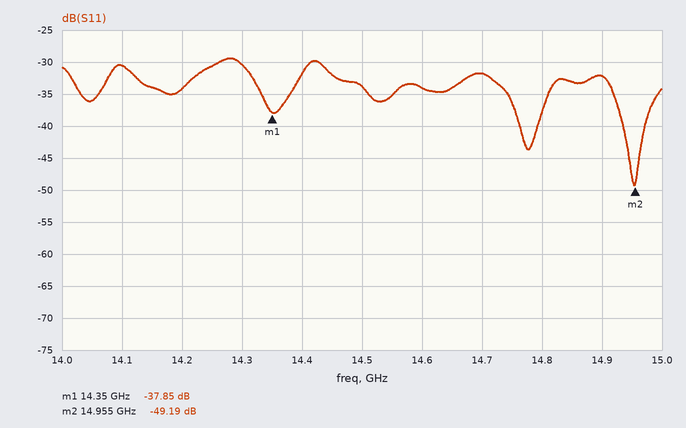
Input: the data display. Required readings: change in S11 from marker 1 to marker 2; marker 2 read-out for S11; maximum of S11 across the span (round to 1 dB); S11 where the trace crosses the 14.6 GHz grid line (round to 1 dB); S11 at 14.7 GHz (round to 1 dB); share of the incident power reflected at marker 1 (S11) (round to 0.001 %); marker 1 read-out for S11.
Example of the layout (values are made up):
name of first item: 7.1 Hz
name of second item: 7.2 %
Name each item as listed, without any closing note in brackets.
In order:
change in S11 from marker 1 to marker 2: -11.34 dB
marker 2 read-out for S11: -49.19 dB
maximum of S11 across the span: -29 dB
S11 where the trace crosses the 14.6 GHz grid line: -34 dB
S11 at 14.7 GHz: -32 dB
share of the incident power reflected at marker 1 (S11): 0.016 %
marker 1 read-out for S11: -37.85 dB
